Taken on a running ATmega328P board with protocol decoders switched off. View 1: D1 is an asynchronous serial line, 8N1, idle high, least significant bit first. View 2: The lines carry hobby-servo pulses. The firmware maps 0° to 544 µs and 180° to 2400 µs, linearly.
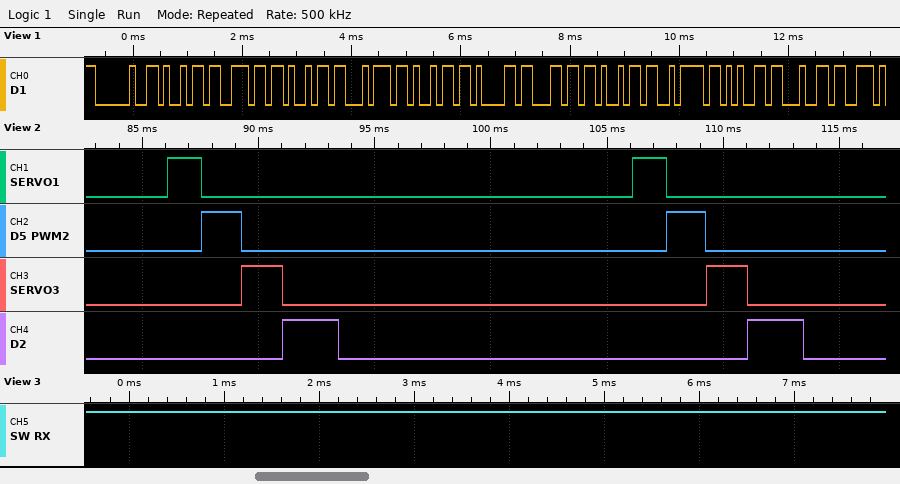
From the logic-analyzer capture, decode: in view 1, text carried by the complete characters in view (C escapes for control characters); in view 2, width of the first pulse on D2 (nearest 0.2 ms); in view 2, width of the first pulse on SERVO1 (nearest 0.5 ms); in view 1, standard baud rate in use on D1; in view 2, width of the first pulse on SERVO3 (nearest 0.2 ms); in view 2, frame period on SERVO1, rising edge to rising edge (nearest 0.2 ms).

" initialized"
2.4 ms
1.5 ms
9600 baud
1.8 ms
20.0 ms
